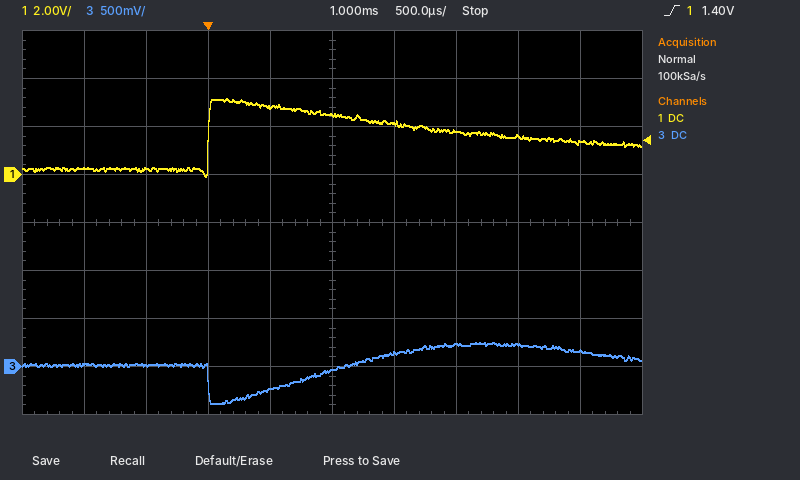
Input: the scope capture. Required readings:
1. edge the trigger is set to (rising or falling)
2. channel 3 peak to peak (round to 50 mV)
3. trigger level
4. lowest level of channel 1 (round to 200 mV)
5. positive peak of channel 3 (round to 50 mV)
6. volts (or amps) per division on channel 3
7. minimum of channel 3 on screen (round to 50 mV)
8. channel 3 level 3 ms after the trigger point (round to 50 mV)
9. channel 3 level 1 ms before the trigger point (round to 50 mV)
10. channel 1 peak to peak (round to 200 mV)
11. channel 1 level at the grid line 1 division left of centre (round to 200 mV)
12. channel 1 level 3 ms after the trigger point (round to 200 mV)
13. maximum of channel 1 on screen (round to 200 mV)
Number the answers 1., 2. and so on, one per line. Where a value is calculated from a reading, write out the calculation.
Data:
1. rising
2. 250 mV − (-400 mV) = 650 mV
3. 1.40 V
4. 0.0 V
5. 250 mV
6. 500 mV
7. -400 mV
8. 150 mV
9. 0 mV
10. 3.2 V − (0.0 V) = 3.2 V
11. 2.8 V
12. 1.4 V
13. 3.2 V
